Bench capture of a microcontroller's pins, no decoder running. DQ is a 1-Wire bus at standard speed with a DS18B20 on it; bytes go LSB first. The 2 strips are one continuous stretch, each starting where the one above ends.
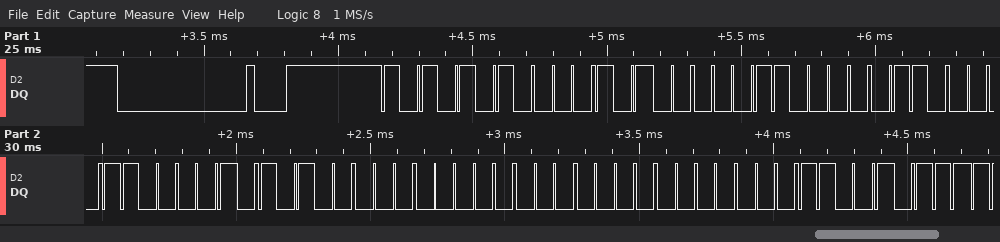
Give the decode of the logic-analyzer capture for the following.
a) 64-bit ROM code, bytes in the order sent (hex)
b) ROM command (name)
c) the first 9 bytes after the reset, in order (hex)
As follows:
28 18 0C 43 05 00 00 98
Match ROM
55 28 18 0C 43 05 00 00 98
